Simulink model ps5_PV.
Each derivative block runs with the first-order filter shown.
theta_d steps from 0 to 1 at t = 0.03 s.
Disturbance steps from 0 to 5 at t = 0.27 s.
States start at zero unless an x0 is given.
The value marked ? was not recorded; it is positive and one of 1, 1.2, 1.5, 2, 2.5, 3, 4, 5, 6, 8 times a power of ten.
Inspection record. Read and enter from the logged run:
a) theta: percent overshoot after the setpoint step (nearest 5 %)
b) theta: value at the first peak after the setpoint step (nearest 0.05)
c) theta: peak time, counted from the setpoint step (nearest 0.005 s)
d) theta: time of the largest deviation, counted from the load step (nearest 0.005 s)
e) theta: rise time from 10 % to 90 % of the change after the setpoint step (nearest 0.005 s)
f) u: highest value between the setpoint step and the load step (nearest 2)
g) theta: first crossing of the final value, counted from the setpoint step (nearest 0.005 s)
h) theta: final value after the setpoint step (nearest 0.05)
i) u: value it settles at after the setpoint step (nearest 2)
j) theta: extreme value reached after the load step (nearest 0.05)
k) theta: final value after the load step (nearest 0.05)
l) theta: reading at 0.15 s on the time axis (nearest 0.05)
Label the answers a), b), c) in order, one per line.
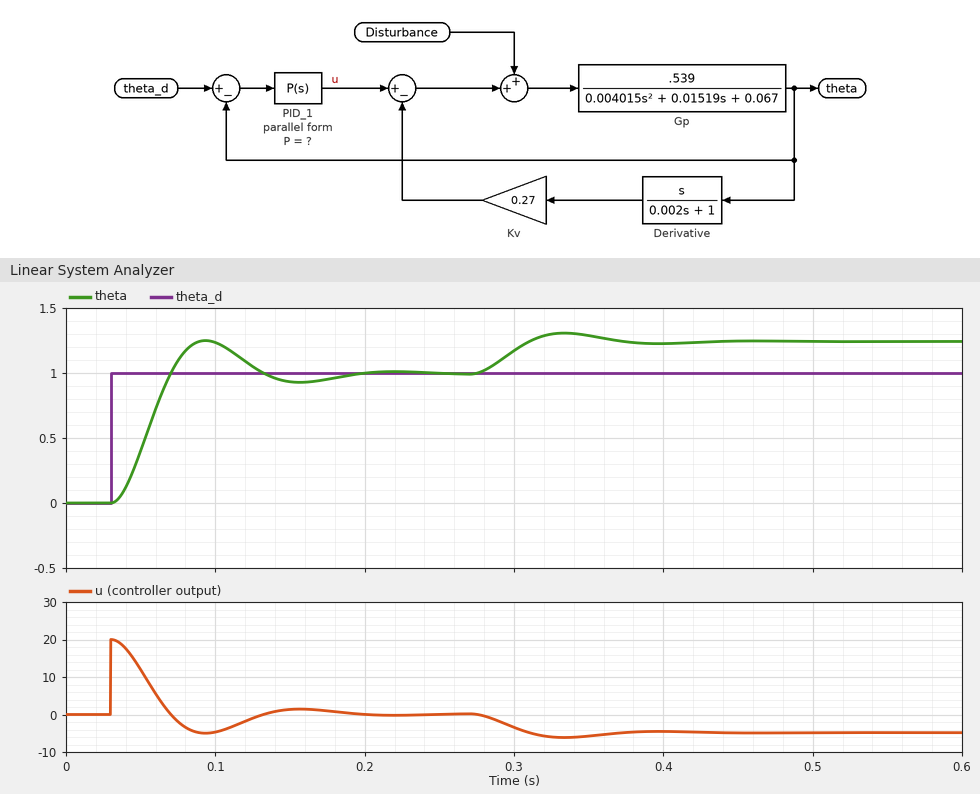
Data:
a) 25 %
b) 1.25
c) 0.065 s
d) 0.065 s
e) 0.025 s
f) 20
g) 0.040 s
h) 1.00
i) 0
j) 1.30
k) 1.25
l) 0.95
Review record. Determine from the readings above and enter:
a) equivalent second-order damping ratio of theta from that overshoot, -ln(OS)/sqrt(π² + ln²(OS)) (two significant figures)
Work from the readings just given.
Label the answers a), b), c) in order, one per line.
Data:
a) 0.40
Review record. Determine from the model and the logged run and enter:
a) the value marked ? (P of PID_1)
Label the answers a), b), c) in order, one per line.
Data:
a) 20
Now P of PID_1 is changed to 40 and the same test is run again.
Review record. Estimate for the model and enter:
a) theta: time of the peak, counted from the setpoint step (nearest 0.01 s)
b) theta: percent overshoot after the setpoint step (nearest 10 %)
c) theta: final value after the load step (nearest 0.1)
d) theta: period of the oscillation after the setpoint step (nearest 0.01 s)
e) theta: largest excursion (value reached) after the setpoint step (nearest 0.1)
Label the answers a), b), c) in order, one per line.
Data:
a) 0.04 s
b) 40 %
c) 1.1
d) 0.09 s
e) 1.4
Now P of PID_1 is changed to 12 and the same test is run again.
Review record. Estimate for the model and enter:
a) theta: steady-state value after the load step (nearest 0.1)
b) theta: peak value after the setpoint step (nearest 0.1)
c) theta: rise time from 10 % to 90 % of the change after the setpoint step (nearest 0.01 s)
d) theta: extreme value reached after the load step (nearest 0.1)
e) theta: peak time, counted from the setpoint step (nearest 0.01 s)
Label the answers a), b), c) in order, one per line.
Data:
a) 1.4
b) 1.1
c) 0.04 s
d) 1.5
e) 0.09 s
